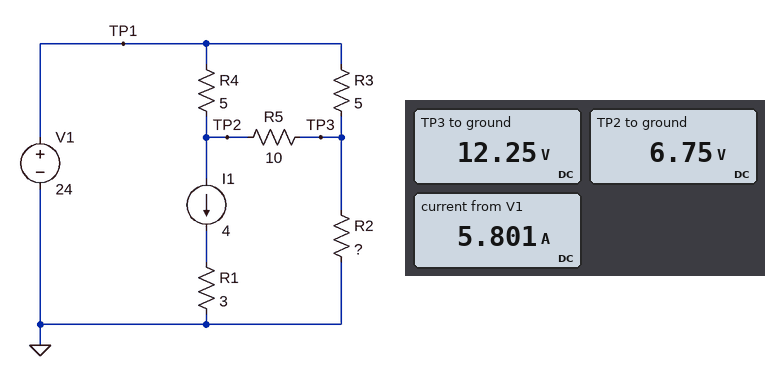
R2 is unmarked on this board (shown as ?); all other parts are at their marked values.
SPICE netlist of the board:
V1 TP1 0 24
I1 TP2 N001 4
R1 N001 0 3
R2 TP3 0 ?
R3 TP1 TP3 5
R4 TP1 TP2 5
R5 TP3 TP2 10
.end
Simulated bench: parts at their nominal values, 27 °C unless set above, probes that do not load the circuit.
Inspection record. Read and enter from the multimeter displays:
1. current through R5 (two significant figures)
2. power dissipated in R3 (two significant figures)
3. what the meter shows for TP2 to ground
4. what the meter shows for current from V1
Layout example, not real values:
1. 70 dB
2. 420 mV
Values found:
1. 550 mA
2. 28 W
3. 6.75 V
4. 5.801 A
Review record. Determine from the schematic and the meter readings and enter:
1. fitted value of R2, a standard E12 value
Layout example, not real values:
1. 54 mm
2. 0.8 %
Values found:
1. 6.8 Ω
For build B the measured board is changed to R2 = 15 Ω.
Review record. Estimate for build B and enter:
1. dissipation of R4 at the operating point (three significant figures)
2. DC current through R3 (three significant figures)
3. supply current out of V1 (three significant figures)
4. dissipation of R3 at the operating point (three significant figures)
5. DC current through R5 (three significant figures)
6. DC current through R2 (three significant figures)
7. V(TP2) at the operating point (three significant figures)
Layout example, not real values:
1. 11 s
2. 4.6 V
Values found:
1. 52.9 W
2. 1.76 A
3. 5.01 A
4. 15.5 W
5. 747 mA
6. 1.01 A
7. 7.73 V
